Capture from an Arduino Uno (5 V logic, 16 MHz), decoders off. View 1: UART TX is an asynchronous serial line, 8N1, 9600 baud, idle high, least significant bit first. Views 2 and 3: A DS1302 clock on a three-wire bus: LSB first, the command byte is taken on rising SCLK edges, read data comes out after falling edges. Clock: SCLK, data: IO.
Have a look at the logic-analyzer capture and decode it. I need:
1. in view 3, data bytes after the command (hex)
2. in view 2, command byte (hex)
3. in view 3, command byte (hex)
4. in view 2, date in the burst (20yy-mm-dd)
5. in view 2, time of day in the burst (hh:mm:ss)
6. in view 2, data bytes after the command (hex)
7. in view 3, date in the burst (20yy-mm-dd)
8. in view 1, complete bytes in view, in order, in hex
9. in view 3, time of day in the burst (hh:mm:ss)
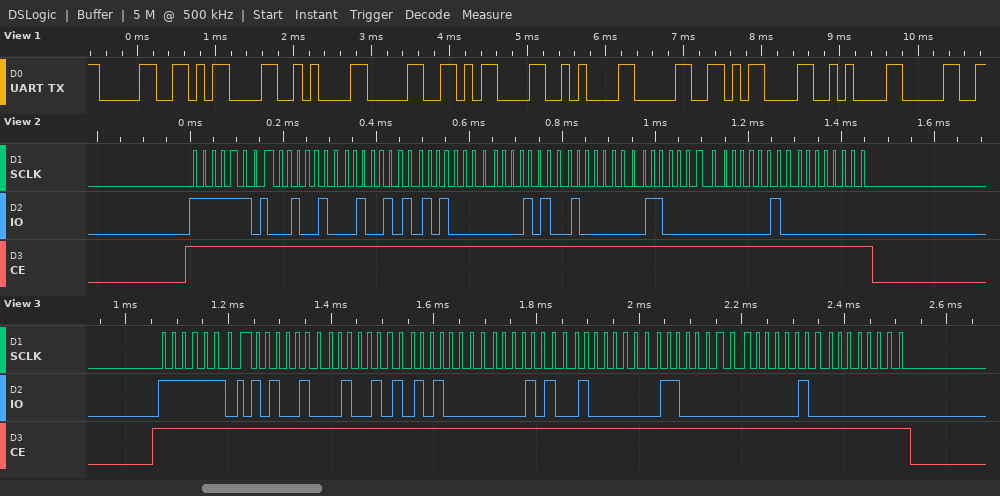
25 52 05 28 01 03 20 00
0xBF
0xBF
2020-01-28
05:52:24
24 52 05 28 01 03 20 00
2020-01-28
30 0D 0A 30 0D 0A 30 0D 0A 30
05:52:25
